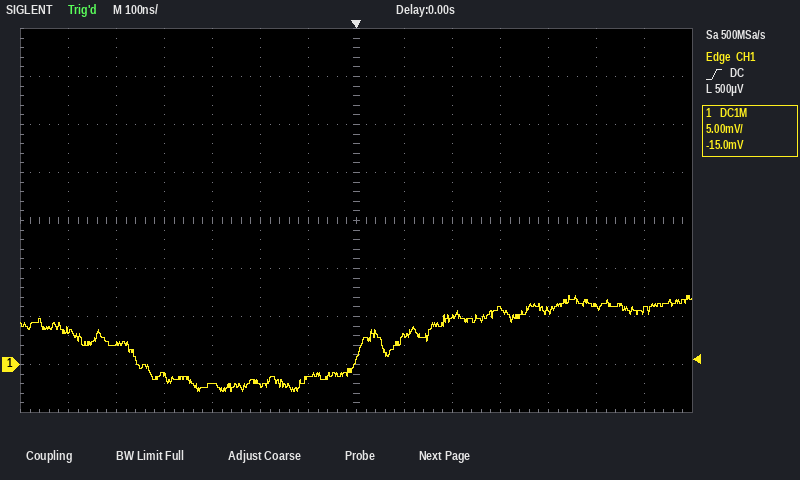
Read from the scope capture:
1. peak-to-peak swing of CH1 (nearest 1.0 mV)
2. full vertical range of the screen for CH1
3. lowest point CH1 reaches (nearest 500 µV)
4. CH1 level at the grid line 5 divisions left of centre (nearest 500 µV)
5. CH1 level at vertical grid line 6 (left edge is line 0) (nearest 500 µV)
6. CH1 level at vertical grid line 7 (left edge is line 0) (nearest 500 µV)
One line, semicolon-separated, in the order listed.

10.0 mV; 40 mV; -3.0 mV; 2.0 mV; -1.5 mV; 500 µV
